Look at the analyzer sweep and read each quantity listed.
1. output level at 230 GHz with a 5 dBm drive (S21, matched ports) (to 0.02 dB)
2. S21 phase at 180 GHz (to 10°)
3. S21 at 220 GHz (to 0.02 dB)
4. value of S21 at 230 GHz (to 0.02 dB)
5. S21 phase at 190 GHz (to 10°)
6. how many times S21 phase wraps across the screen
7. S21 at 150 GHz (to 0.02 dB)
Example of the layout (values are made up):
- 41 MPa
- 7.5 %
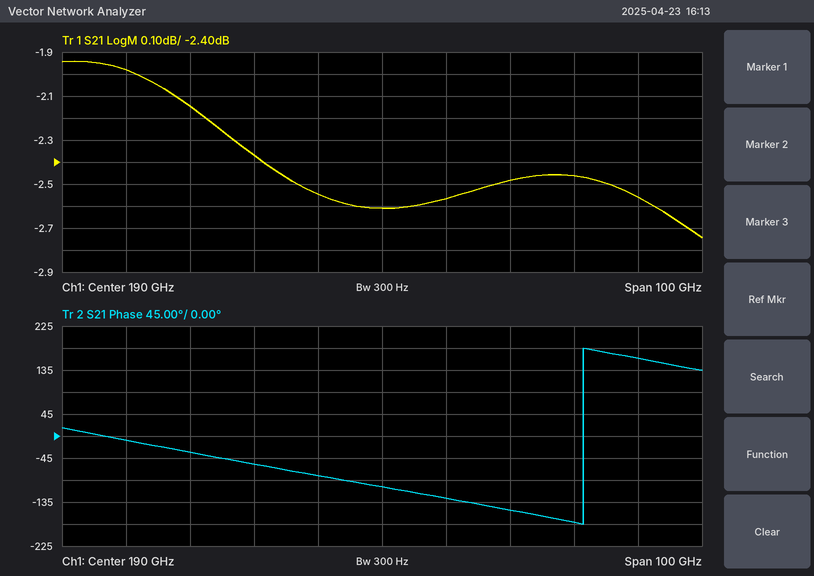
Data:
- 2.44 dBm
- -80°
- -2.46 dB
- -2.56 dB
- -100°
- 1
- -1.98 dB
